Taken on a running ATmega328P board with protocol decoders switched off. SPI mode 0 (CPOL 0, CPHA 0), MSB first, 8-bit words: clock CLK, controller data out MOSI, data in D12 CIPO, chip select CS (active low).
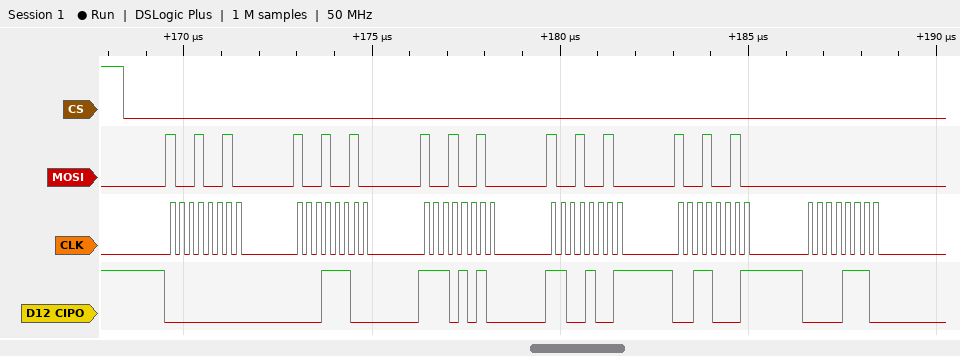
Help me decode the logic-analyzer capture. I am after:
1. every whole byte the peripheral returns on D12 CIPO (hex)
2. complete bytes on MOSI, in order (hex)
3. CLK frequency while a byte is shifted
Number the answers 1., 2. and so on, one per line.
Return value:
1. 00 1C EA C9 31 0E
2. 92 92 92 92 92 00
3. 4 MHz
